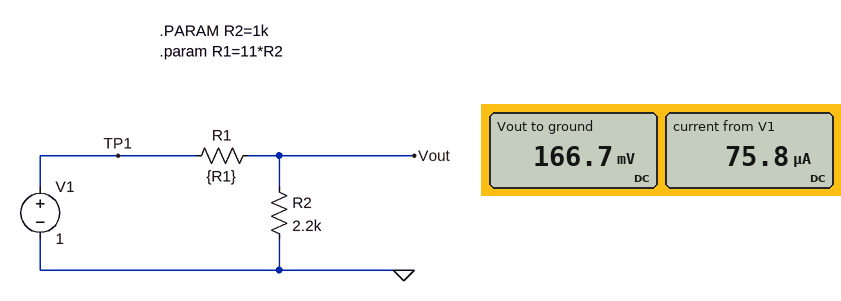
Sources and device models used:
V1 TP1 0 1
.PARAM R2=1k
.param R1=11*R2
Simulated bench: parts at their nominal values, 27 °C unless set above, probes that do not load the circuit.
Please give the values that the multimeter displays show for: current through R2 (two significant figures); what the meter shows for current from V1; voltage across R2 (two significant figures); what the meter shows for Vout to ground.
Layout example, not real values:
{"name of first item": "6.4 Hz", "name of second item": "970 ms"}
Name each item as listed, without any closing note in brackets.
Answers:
{"current through R2": "76 µA", "what the meter shows for current from V1": "75.8 µA", "voltage across R2": "170 mV", "what the meter shows for Vout to ground": "166.7 mV"}
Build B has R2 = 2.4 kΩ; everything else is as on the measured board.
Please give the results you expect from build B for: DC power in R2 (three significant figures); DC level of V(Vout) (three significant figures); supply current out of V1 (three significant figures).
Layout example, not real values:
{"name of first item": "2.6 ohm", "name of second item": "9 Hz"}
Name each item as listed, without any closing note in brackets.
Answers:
{"DC power in R2": "13.4 µW", "DC level of V(Vout)": "179 mV", "supply current out of V1": "74.6 µA"}
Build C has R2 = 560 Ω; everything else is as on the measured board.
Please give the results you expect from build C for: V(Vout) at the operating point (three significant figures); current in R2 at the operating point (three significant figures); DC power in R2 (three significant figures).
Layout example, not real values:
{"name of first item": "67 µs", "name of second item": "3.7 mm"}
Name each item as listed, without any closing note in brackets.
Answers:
{"V(Vout) at the operating point": "48.4 mV", "current in R2 at the operating point": "86.5 µA", "DC power in R2": "4.19 µW"}
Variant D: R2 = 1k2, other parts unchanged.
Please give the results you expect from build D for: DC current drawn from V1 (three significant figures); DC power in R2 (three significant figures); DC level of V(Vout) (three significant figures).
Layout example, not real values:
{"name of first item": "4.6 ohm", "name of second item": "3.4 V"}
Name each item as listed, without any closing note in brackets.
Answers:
{"DC current drawn from V1": "82.0 µA", "DC power in R2": "8.06 µW", "DC level of V(Vout)": "98.4 mV"}
